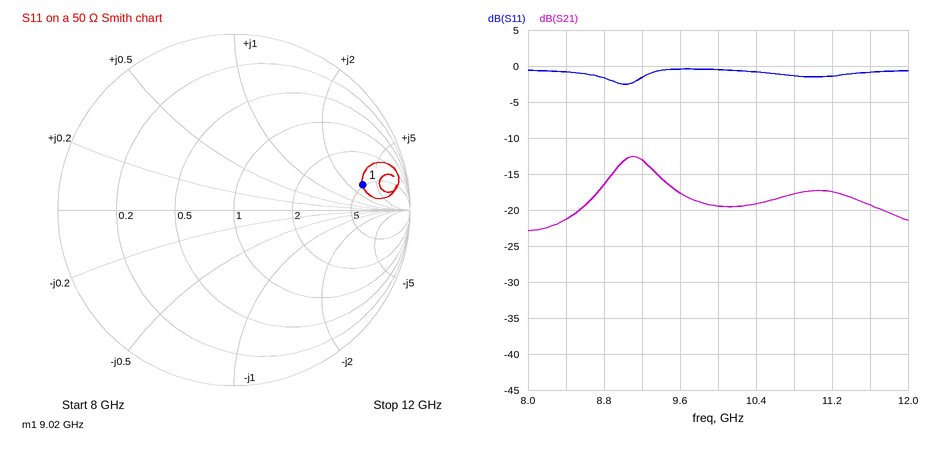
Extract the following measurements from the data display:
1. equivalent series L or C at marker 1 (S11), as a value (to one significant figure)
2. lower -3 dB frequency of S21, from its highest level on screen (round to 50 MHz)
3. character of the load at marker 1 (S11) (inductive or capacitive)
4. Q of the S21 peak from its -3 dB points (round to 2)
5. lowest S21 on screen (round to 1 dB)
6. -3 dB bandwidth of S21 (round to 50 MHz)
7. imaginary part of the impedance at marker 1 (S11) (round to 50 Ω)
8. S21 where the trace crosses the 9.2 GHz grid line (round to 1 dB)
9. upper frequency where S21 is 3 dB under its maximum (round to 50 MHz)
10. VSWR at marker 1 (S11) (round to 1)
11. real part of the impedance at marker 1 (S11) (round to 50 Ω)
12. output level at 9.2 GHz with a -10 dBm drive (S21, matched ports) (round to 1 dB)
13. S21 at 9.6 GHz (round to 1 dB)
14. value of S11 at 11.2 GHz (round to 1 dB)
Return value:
3 nH
8.85 GHz
inductive
16
-23 dB
550 MHz
+150 Ω
-13 dB
9.40 GHz
7
250 Ω
-23 dBm
-18 dB
-1 dB
